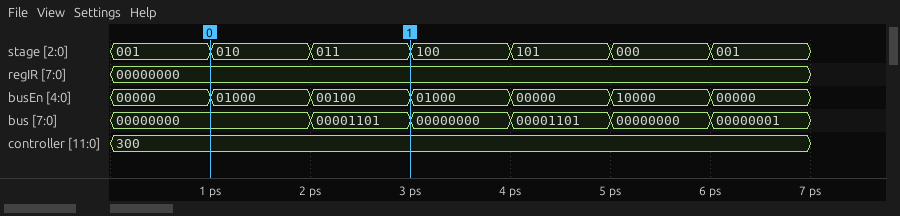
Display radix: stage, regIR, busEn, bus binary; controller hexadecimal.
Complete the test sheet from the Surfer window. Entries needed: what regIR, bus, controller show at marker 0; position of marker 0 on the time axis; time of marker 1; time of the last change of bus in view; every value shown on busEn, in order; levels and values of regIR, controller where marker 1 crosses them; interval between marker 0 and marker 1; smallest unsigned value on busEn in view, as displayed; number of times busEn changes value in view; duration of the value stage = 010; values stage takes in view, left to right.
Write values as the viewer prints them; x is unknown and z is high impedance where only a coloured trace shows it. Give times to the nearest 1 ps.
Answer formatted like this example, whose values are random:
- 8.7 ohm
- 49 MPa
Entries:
- regIR=00000000, bus=00000000, controller=300
- 1 ps
- 3 ps
- 6 ps
- 00000, 01000, 00100, 01000, 00000, 10000, 00000
- regIR=00000000, controller=300
- 2 ps
- 00000
- 6
- 1 ps
- 001, 010, 011, 100, 101, 000, 001
